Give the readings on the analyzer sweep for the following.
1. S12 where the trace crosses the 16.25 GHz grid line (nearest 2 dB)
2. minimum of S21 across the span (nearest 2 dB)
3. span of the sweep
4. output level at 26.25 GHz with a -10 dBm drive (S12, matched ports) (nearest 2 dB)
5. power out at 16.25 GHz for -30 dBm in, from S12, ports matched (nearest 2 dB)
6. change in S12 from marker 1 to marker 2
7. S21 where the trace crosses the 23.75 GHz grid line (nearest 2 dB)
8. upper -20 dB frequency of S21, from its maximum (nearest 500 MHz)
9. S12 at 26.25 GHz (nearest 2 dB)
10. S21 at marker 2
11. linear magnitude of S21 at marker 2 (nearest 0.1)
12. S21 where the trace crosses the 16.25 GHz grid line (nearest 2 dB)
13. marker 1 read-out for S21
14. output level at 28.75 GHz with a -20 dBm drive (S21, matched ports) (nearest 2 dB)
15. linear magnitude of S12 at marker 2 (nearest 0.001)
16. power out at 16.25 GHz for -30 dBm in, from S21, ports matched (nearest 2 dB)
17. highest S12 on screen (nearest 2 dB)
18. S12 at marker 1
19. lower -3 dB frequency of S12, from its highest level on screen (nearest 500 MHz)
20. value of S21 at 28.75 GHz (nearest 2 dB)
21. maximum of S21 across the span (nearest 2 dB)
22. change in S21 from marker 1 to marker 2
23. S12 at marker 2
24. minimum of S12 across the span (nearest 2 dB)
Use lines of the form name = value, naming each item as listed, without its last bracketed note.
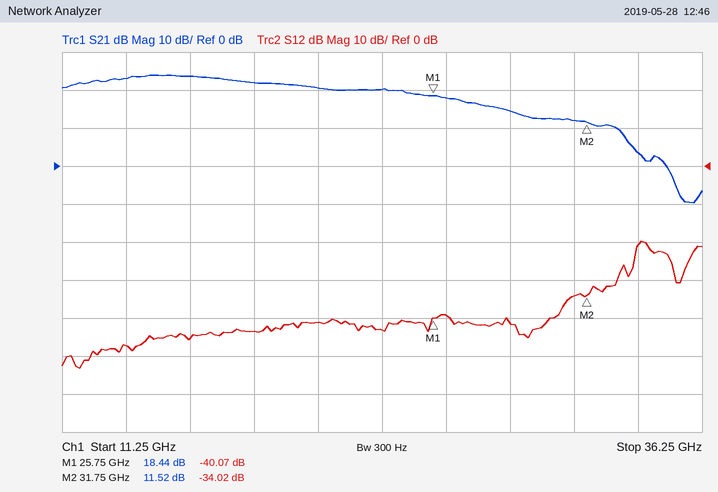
S12 where the trace crosses the 16.25 GHz grid line = -46 dB
minimum of S21 across the span = -10 dB
span of the sweep = 25 GHz
output level at 26.25 GHz with a -10 dBm drive (S12, matched ports) = -50 dBm
power out at 16.25 GHz for -30 dBm in, from S12, ports matched = -76 dBm
change in S12 from marker 1 to marker 2 = 6.05 dB
S21 where the trace crosses the 23.75 GHz grid line = 20 dB
upper -20 dB frequency of S21, from its maximum = 33.5 GHz
S12 at 26.25 GHz = -40 dB
S21 at marker 2 = 11.52 dB
linear magnitude of S21 at marker 2 = 3.8
S21 where the trace crosses the 16.25 GHz grid line = 24 dB
marker 1 read-out for S21 = 18.44 dB
output level at 28.75 GHz with a -20 dBm drive (S21, matched ports) = -6 dBm
linear magnitude of S12 at marker 2 = 0.020
power out at 16.25 GHz for -30 dBm in, from S21, ports matched = -6 dBm
highest S12 on screen = -20 dB
S12 at marker 1 = -40.07 dB
lower -3 dB frequency of S12, from its highest level on screen = 33.5 GHz
value of S21 at 28.75 GHz = 14 dB
maximum of S21 across the span = 24 dB
change in S21 from marker 1 to marker 2 = -6.92 dB
S12 at marker 2 = -34.02 dB
minimum of S12 across the span = -54 dB
